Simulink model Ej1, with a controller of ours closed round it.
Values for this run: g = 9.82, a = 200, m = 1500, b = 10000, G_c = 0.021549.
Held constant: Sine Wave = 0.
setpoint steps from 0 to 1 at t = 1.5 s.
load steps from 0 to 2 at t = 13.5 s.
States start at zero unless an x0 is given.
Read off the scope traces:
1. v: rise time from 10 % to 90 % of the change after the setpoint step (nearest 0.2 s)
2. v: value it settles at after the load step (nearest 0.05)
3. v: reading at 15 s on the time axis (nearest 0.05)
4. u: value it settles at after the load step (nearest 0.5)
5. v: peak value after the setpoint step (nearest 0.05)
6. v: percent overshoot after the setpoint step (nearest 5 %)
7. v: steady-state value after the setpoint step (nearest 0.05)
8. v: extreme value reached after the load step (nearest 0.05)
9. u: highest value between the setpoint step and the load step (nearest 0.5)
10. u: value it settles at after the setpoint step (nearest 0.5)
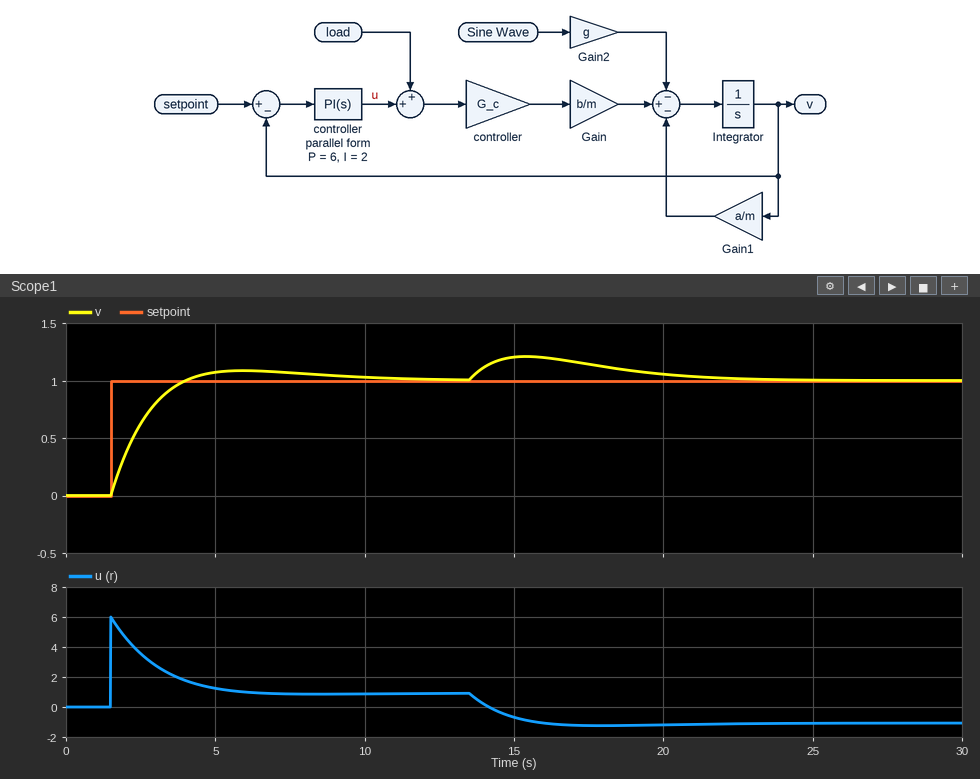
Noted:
1.8 s
1.00
1.20
-1.0
1.10
10 %
1.00
1.20
6.0
1.0
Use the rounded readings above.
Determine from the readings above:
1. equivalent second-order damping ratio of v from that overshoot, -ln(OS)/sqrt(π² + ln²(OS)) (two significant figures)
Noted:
0.59
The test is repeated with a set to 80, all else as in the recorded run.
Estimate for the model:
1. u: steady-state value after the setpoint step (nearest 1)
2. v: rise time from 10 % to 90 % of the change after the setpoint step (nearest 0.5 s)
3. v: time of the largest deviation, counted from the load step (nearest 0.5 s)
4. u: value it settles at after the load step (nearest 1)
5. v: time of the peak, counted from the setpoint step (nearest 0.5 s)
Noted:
0
1.5 s
2.0 s
-2
4.0 s
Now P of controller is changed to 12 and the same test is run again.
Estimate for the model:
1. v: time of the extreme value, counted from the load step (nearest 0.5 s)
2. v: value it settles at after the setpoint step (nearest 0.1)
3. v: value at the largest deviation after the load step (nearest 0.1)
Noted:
1.5 s
1.0
1.1
